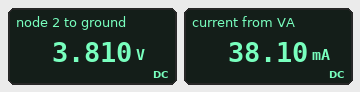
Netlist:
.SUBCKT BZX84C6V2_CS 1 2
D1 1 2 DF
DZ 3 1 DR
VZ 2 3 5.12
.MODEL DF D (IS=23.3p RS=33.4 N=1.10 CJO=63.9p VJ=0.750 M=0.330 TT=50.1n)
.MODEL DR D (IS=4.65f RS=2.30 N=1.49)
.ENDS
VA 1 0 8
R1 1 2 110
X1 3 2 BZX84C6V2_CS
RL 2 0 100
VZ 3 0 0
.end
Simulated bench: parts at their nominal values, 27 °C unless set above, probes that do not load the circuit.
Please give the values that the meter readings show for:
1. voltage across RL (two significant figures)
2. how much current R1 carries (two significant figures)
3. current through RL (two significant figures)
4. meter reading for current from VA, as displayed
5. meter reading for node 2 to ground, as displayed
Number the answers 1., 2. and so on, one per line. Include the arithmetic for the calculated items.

1. 3.81 V = 3.8 V
2. (8 V - 3.81 V) / 110 Ω = 38 mA
3. (3.81 V) / 100 Ω = 38 mA
4. 38.10 mA
5. 3.810 V
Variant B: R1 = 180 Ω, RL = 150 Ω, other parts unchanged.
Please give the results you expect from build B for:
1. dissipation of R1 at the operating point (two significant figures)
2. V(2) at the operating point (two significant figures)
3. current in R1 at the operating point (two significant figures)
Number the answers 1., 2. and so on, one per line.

1. 110 mW
2. 3.6 V
3. 24 mA
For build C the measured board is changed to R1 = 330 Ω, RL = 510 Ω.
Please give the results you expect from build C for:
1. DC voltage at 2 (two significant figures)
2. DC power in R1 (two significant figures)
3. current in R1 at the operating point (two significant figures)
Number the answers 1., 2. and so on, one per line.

1. 4.9 V
2. 30 mW
3. 9.5 mA
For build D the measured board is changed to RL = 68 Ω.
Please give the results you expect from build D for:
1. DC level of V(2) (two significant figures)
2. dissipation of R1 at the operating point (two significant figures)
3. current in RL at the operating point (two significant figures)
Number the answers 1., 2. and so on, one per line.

1. 3.1 V
2. 220 mW
3. 45 mA
